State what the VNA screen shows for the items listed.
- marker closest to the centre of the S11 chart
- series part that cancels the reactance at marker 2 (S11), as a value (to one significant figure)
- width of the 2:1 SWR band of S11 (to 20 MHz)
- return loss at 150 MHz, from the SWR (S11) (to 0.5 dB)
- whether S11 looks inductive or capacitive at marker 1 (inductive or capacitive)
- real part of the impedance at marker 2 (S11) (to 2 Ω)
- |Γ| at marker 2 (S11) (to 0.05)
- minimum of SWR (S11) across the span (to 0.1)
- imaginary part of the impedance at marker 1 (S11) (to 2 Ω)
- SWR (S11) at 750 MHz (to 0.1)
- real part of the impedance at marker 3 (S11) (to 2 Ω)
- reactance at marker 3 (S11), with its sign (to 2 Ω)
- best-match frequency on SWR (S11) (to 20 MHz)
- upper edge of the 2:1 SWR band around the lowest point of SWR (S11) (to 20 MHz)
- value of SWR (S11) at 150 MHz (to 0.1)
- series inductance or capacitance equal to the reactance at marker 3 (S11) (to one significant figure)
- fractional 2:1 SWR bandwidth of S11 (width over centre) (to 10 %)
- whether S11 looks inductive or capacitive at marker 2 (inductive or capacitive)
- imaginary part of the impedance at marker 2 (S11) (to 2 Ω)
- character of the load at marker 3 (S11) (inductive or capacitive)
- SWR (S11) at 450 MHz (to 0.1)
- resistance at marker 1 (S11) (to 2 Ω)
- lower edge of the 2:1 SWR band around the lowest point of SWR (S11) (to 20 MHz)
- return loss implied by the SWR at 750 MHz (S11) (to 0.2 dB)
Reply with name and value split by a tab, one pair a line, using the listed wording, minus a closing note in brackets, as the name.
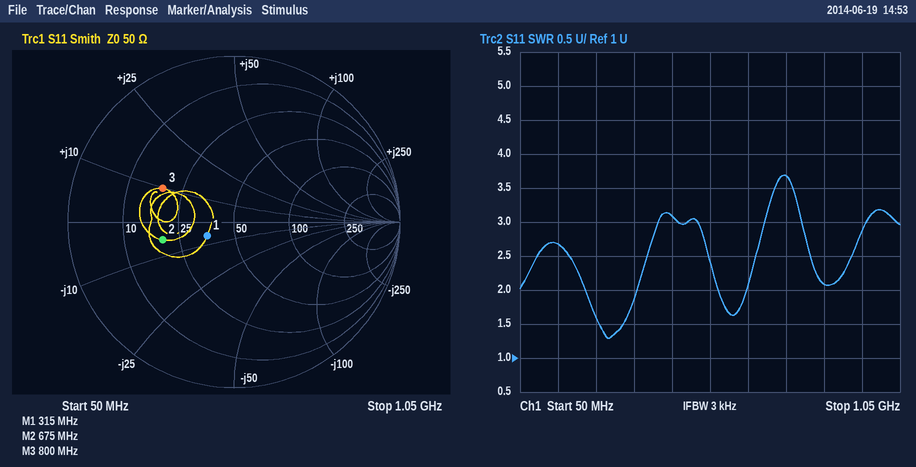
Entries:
marker closest to the centre of the S11 chart	marker 1
series part that cancels the reactance at marker 2 (S11), as a value	1 nH
width of the 2:1 SWR band of S11	140 MHz
return loss at 150 MHz, from the SWR (S11)	7.0 dB
whether S11 looks inductive or capacitive at marker 1	capacitive
real part of the impedance at marker 2 (S11)	20 Ω
|Γ| at marker 2 (S11)	0.45
minimum of SWR (S11) across the span	1.3
imaginary part of the impedance at marker 1 (S11)	-6 Ω
SWR (S11) at 750 MHz	3.7
real part of the impedance at marker 3 (S11)	18 Ω
reactance at marker 3 (S11), with its sign	+10 Ω
best-match frequency on SWR (S11)	280 MHz
upper edge of the 2:1 SWR band around the lowest point of SWR (S11)	360 MHz
value of SWR (S11) at 150 MHz	2.7
series inductance or capacitance equal to the reactance at marker 3 (S11)	2 nH
fractional 2:1 SWR bandwidth of S11 (width over centre)	50 %
whether S11 looks inductive or capacitive at marker 2	capacitive
imaginary part of the impedance at marker 2 (S11)	-6 Ω
character of the load at marker 3 (S11)	inductive
SWR (S11) at 450 MHz	3.1
resistance at marker 1 (S11)	36 Ω
lower edge of the 2:1 SWR band around the lowest point of SWR (S11)	220 MHz
return loss implied by the SWR at 750 MHz (S11)	4.8 dB
